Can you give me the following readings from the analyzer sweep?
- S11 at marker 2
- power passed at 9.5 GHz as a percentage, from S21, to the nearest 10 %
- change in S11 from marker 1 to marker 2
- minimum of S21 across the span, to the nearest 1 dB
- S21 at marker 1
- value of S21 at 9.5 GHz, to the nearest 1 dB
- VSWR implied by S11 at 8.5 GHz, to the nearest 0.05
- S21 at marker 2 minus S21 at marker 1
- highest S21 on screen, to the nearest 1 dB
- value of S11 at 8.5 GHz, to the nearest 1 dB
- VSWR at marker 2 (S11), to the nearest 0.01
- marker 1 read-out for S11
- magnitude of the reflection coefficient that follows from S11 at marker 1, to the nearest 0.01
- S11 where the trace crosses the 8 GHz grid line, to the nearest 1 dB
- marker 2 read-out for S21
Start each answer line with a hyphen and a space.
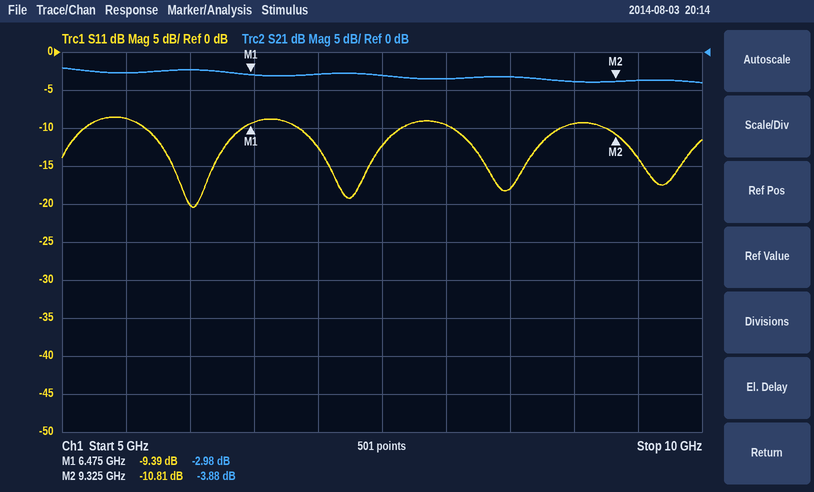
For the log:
- -10.81 dB
- 40 %
- -1.42 dB
- -4 dB
- -2.98 dB
- -4 dB
- 1.30
- -0.90 dB
- -2 dB
- -18 dB
- 1.81
- -9.39 dB
- 0.34
- -10 dB
- -3.88 dB
